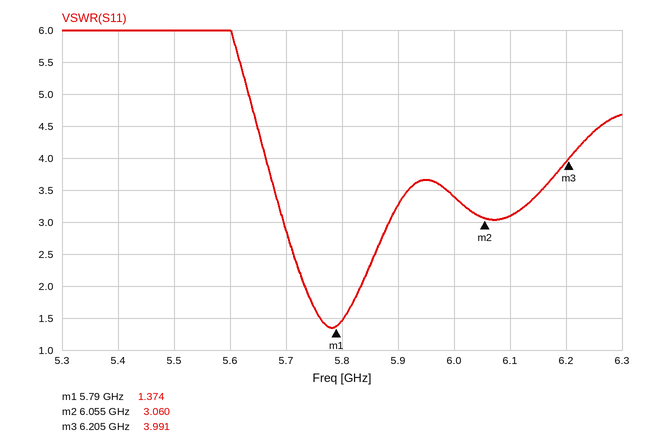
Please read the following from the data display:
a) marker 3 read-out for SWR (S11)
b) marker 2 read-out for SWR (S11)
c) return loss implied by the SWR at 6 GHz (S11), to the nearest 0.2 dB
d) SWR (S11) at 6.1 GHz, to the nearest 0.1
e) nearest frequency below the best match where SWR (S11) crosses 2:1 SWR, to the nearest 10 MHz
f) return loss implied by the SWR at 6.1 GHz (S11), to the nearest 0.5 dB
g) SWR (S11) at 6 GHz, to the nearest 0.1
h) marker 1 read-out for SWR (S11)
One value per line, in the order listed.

3.991
3.060
5.2 dB
3.1
5.73 GHz
6.0 dB
3.4
1.374
